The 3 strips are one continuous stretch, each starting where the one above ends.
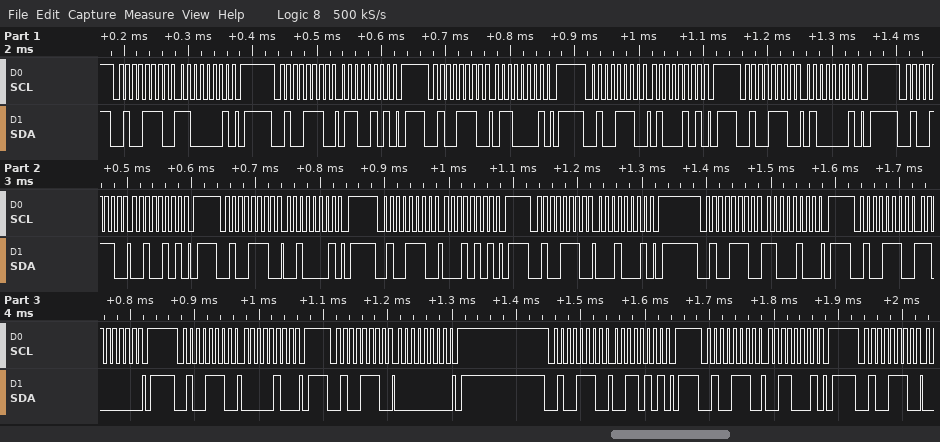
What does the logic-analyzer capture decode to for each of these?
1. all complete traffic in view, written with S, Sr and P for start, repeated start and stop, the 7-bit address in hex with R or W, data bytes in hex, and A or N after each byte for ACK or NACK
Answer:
S 27W A C1 A P S 27W A 65 A P S 27W A 61 A P S 27W A 45 A P S 27W A 41 A P S 27W A 25 A P S 27W A 21 A P S 27W A 15 A P S 27W A 11 A P S 27W A C4 A P S 27W A C0 A P S 27W A 04 A P S 27W A 00 A P S 27W A 35 A P S 27W A 31 A P S 27W A
